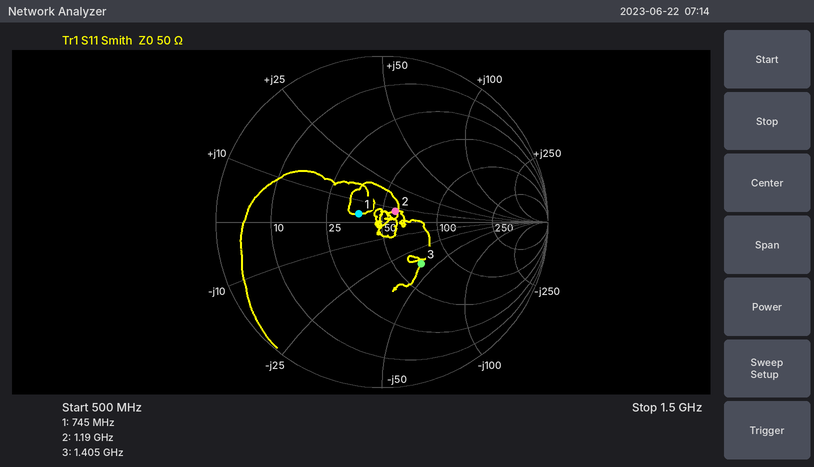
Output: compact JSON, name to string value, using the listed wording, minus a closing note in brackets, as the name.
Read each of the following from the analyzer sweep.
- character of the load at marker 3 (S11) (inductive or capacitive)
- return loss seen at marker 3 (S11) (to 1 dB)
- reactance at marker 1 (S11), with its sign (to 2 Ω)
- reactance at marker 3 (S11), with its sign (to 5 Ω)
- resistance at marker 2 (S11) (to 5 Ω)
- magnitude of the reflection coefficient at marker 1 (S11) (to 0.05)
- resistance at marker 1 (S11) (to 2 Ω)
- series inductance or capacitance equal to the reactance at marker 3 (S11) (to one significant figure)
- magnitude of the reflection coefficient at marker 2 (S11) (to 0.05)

{"character of the load at marker 3 (S11)": "capacitive", "return loss seen at marker 3 (S11)": "9 dB", "reactance at marker 1 (S11), with its sign": "+4 Ω", "reactance at marker 3 (S11), with its sign": "-40 Ω", "resistance at marker 2 (S11)": "60 Ω", "magnitude of the reflection coefficient at marker 1 (S11)": "0.15", "resistance at marker 1 (S11)": "38 Ω", "series inductance or capacitance equal to the reactance at marker 3 (S11)": "3 pF", "magnitude of the reflection coefficient at marker 2 (S11)": "0.10"}
